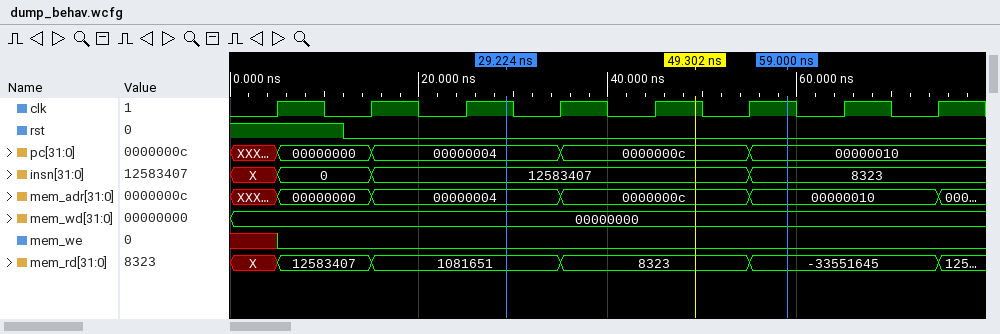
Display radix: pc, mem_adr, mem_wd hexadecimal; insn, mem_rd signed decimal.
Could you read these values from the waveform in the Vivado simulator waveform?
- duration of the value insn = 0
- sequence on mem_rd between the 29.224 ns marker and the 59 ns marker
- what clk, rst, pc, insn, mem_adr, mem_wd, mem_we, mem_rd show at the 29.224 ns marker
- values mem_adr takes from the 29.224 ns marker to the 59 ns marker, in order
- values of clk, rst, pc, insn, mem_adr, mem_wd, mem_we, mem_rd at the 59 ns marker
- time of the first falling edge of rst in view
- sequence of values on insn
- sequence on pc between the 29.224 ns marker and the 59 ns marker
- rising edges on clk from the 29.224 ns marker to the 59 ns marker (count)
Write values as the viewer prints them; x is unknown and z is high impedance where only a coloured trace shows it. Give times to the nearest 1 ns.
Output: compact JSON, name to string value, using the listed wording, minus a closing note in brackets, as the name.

{"duration of the value insn = 0": "10 ns", "sequence on mem_rd between the 29.224 ns marker and the 59 ns marker": "1081651, 8323, -33551645", "what clk, rst, pc, insn, mem_adr, mem_wd, mem_we, mem_rd show at the 29.224 ns marker": "clk=1, rst=0, pc=00000004, insn=12583407, mem_adr=00000004, mem_wd=00000000, mem_we=0, mem_rd=1081651", "values mem_adr takes from the 29.224 ns marker to the 59 ns marker, in order": "00000004, 0000000c, 00000010", "values of clk, rst, pc, insn, mem_adr, mem_wd, mem_we, mem_rd at the 59 ns marker": "clk=1, rst=0, pc=00000010, insn=8323, mem_adr=00000010, mem_wd=00000000, mem_we=0, mem_rd=-33551645", "time of the first falling edge of rst in view": "12 ns", "sequence of values on insn": "X, 0, 12583407, 8323", "sequence on pc between the 29.224 ns marker and the 59 ns marker": "00000004, 0000000c, 00000010", "rising edges on clk from the 29.224 ns marker to the 59 ns marker": "3"}
